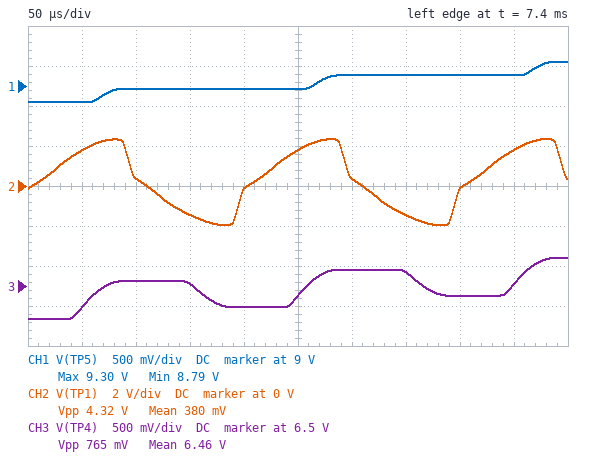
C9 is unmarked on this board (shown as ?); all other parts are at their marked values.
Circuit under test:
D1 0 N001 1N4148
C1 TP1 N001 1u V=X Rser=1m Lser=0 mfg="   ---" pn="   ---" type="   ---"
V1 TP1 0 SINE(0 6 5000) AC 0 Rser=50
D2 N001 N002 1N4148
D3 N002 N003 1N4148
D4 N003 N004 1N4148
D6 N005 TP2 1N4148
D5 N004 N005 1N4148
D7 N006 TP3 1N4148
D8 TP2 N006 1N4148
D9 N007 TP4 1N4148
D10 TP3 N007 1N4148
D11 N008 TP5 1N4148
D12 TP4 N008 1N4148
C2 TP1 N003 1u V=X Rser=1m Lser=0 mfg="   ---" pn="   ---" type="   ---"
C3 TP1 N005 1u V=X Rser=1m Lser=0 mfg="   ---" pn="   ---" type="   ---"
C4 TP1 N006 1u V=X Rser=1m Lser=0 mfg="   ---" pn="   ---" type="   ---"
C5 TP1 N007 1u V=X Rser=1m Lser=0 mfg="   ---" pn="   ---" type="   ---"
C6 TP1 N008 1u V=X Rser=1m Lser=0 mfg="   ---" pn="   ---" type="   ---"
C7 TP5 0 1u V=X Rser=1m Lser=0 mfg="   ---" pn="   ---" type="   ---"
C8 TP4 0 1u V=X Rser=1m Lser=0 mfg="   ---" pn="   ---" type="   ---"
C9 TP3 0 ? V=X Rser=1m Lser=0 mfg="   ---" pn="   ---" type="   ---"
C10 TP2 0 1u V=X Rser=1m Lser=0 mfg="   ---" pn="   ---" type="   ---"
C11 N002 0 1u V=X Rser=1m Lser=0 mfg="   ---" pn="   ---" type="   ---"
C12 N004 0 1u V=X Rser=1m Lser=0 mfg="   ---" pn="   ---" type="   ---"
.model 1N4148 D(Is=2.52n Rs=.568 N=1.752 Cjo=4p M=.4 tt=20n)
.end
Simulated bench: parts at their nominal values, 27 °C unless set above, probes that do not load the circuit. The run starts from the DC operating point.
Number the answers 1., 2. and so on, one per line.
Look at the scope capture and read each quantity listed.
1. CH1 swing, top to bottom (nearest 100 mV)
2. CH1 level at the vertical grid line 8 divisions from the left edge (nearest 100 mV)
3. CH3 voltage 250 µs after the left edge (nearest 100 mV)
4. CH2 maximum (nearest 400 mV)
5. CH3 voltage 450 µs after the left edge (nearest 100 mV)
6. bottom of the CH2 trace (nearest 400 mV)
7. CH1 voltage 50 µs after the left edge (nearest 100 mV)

1. 500 mV
2. 9.1 V
3. 6.4 V
4. 2.4 V
5. 6.5 V
6. -2.0 V
7. 8.8 V
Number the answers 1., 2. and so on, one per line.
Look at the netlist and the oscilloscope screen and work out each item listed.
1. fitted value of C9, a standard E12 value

1. 1.8 µF
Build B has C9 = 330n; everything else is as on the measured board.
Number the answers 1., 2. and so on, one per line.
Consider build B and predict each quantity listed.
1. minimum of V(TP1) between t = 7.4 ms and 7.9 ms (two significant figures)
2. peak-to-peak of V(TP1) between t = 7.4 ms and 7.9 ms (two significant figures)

1. -2.1 V
2. 4.6 V
